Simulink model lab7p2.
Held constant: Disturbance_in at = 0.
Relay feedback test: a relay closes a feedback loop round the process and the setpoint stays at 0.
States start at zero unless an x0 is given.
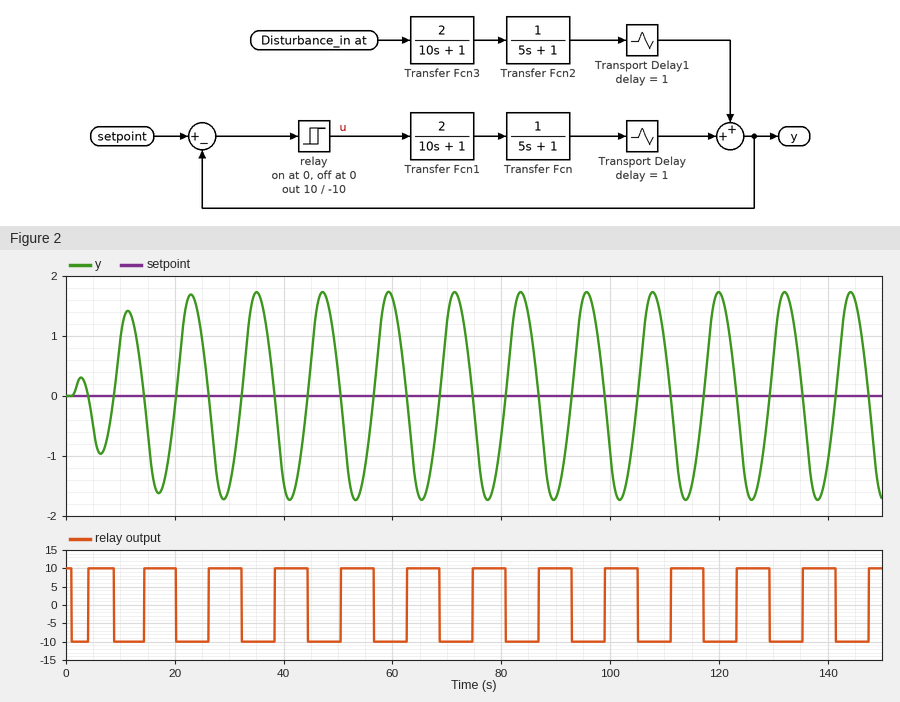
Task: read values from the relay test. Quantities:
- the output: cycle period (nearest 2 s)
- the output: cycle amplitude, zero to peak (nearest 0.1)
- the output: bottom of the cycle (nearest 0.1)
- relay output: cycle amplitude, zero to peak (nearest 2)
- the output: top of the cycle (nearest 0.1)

12 s
1.7
-1.7
10
1.7
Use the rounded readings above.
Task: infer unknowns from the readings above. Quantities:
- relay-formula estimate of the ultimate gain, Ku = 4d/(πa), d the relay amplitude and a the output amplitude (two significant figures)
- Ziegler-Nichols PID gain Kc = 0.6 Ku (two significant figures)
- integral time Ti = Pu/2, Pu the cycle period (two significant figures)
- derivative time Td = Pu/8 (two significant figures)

7.5
4.5
6.0 s
1.5 s
